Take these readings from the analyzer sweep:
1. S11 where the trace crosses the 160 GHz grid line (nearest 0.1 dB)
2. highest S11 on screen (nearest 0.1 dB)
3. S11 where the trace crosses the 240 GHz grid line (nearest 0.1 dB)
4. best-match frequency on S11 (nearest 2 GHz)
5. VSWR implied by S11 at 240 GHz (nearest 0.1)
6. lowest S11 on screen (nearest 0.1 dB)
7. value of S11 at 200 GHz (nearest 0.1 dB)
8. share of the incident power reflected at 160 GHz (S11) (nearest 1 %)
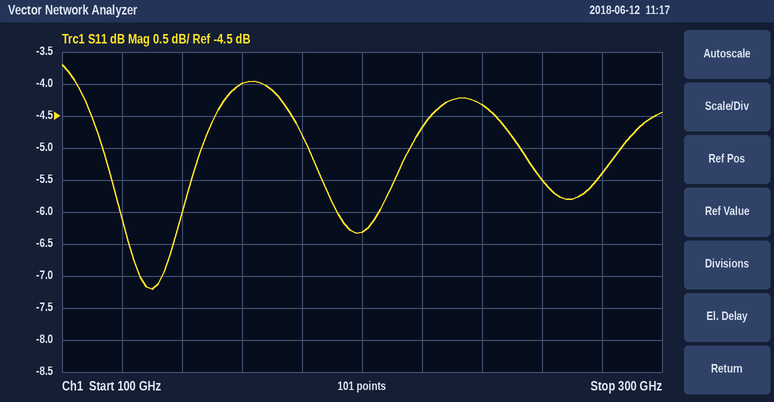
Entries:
-4.0 dB
-3.7 dB
-4.3 dB
130 GHz
4.1
-7.2 dB
-6.3 dB
40 %
